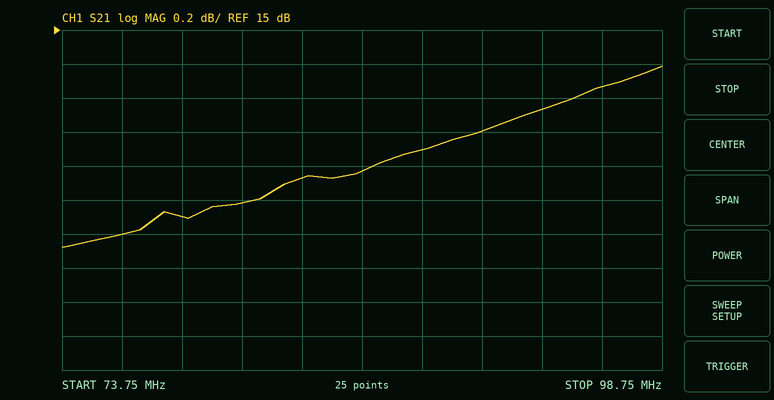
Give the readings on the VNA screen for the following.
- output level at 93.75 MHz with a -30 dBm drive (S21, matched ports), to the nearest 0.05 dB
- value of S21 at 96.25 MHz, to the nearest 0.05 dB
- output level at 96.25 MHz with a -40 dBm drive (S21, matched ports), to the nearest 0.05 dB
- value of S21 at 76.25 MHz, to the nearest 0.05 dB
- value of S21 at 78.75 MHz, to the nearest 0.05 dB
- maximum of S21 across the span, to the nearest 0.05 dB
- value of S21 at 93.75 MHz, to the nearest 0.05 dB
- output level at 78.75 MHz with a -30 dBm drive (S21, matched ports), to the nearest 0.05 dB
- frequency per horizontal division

-15.45 dBm
14.65 dB
-25.35 dBm
13.80 dB
13.90 dB
14.80 dB
14.55 dB
-16.10 dBm
2.5 MHz
